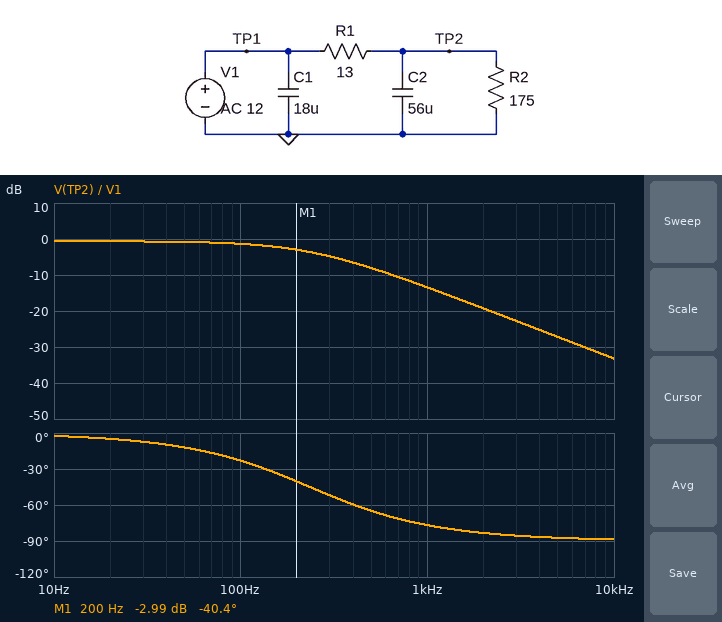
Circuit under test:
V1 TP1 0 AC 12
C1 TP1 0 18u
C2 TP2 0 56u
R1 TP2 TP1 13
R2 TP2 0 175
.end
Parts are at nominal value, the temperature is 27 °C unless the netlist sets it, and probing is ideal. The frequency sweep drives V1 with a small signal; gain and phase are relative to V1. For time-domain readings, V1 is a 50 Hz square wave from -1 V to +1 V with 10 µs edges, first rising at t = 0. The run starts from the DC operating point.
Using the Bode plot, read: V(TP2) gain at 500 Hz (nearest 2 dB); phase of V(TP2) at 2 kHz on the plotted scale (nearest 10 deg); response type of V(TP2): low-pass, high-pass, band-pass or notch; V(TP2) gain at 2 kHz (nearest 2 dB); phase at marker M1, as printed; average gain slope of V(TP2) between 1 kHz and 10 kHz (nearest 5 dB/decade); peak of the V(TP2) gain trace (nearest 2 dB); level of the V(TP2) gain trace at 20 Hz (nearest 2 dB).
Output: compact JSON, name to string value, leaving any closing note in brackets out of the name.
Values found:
{"V(TP2) gain at 500 Hz": "-8 dB", "phase of V(TP2) at 2 kHz on the plotted scale": "-80 deg", "response type of V(TP2): low-pass, high-pass, band-pass or notch": "low-pass", "V(TP2) gain at 2 kHz": "-20 dB", "phase at marker M1, as printed": "-40.4 deg", "average gain slope of V(TP2) between 1 kHz and 10 kHz": "-20 dB/decade", "peak of the V(TP2) gain trace": "0 dB", "level of the V(TP2) gain trace at 20 Hz": "0 dB"}
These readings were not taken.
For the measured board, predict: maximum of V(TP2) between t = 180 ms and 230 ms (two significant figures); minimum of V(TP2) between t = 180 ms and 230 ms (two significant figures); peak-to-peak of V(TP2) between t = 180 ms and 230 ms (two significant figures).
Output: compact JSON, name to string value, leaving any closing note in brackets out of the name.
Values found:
{"maximum of V(TP2) between t = 180 ms and 230 ms": "930 mV", "minimum of V(TP2) between t = 180 ms and 230 ms": "-930 mV", "peak-to-peak of V(TP2) between t = 180 ms and 230 ms": "1.9 V"}
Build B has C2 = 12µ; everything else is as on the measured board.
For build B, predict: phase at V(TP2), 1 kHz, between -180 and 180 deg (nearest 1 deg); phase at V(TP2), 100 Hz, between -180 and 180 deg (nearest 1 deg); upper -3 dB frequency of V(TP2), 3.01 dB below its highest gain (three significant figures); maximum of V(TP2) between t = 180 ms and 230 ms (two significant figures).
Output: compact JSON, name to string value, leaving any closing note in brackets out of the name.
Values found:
{"phase at V(TP2), 1 kHz, between -180 and 180 deg": "-42 deg", "phase at V(TP2), 100 Hz, between -180 and 180 deg": "-5 deg", "upper -3 dB frequency of V(TP2), 3.01 dB below its highest gain": "1.10 kHz", "maximum of V(TP2) between t = 180 ms and 230 ms": "930 mV"}
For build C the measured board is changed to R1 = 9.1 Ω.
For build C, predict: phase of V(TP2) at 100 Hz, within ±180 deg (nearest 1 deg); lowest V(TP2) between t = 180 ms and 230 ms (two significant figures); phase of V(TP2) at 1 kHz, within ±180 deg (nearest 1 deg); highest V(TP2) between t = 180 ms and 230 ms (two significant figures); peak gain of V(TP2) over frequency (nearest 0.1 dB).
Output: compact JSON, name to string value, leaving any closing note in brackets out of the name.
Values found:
{"phase of V(TP2) at 100 Hz, within ±180 deg": "-17 deg", "lowest V(TP2) between t = 180 ms and 230 ms": "-950 mV", "phase of V(TP2) at 1 kHz, within ±180 deg": "-72 deg", "highest V(TP2) between t = 180 ms and 230 ms": "950 mV", "peak gain of V(TP2) over frequency": "-0.4 dB"}
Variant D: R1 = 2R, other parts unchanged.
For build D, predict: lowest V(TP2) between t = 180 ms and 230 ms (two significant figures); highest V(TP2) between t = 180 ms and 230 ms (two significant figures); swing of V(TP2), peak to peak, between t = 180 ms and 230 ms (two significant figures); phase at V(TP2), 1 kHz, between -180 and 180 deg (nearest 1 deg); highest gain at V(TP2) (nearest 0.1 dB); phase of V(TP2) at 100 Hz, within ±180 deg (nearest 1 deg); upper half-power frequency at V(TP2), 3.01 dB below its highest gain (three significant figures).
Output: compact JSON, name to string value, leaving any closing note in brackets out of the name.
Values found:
{"lowest V(TP2) between t = 180 ms and 230 ms": "-990 mV", "highest V(TP2) between t = 180 ms and 230 ms": "990 mV", "swing of V(TP2), peak to peak, between t = 180 ms and 230 ms": "2.0 V", "phase at V(TP2), 1 kHz, between -180 and 180 deg": "-35 deg", "highest gain at V(TP2)": "-0.1 dB", "phase of V(TP2) at 100 Hz, within ±180 deg": "-4 deg", "upper half-power frequency at V(TP2), 3.01 dB below its highest gain": "1.44 kHz"}
